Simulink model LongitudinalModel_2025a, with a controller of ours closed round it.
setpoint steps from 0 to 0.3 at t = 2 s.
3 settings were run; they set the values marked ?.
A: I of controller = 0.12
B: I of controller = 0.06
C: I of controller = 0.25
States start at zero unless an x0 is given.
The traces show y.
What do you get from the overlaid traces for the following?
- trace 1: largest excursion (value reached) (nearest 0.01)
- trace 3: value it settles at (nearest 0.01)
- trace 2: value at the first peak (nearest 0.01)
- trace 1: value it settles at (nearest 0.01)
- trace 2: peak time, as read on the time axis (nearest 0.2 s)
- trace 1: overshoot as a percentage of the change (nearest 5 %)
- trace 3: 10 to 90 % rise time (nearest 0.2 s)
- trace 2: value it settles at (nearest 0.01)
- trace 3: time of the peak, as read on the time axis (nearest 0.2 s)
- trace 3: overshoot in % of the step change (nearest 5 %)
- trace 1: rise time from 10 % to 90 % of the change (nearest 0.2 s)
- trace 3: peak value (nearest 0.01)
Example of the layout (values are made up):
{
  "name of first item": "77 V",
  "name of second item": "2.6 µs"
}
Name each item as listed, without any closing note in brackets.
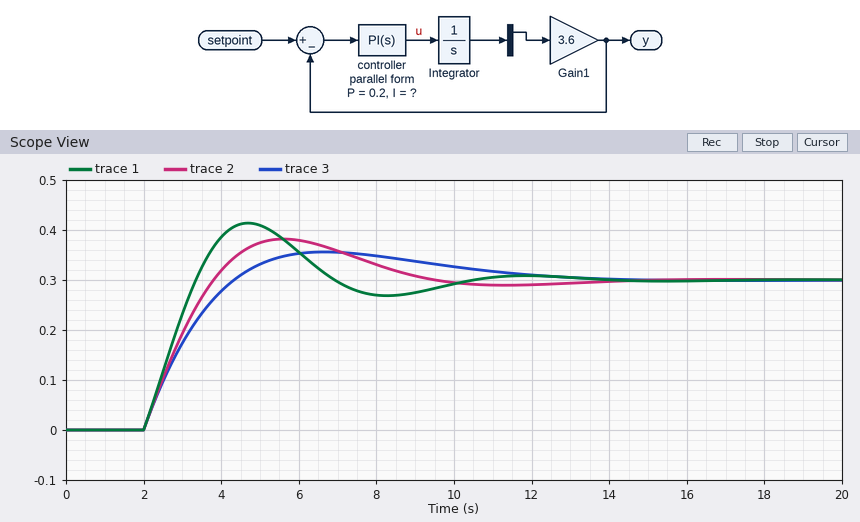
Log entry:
{
  "trace 1: largest excursion (value reached)": "0.41",
  "trace 3: value it settles at": "0.30",
  "trace 2: value at the first peak": "0.38",
  "trace 1: value it settles at": "0.30",
  "trace 2: peak time, as read on the time axis": "5.6 s",
  "trace 1: overshoot as a percentage of the change": "40 %",
  "trace 3: 10 to 90 % rise time": "1.8 s",
  "trace 2: value it settles at": "0.30",
  "trace 3: time of the peak, as read on the time axis": "6.6 s",
  "trace 3: overshoot in % of the step change": "20 %",
  "trace 1: rise time from 10 % to 90 % of the change": "1.0 s",
  "trace 3: peak value": "0.36"
}
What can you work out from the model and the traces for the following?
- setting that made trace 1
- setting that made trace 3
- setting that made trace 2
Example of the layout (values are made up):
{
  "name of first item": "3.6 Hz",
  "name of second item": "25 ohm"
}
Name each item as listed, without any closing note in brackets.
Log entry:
{
  "setting that made trace 1": "C",
  "setting that made trace 3": "B",
  "setting that made trace 2": "A"
}
